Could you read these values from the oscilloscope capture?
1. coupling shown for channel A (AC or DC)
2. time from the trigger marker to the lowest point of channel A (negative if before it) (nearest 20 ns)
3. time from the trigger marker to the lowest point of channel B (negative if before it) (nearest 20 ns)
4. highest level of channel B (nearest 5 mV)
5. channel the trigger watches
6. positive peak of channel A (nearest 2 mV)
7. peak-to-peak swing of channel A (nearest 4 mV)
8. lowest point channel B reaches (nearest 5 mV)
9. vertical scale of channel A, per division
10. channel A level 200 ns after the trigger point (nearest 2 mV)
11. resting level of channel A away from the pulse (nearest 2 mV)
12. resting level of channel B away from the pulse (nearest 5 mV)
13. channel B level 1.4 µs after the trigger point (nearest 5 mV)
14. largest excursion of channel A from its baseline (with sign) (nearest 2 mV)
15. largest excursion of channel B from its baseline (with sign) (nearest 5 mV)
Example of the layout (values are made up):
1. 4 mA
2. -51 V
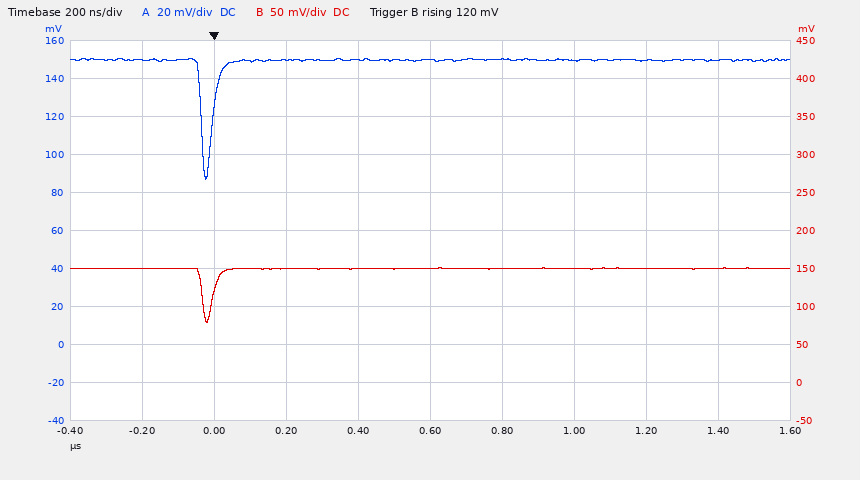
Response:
1. DC
2. -20 ns
3. -20 ns
4. 150 mV
5. channel B
6. 150 mV
7. 64 mV
8. 80 mV
9. 20 mV
10. 150 mV
11. 150 mV
12. 150 mV
13. 150 mV
14. -62 mV
15. -70 mV
